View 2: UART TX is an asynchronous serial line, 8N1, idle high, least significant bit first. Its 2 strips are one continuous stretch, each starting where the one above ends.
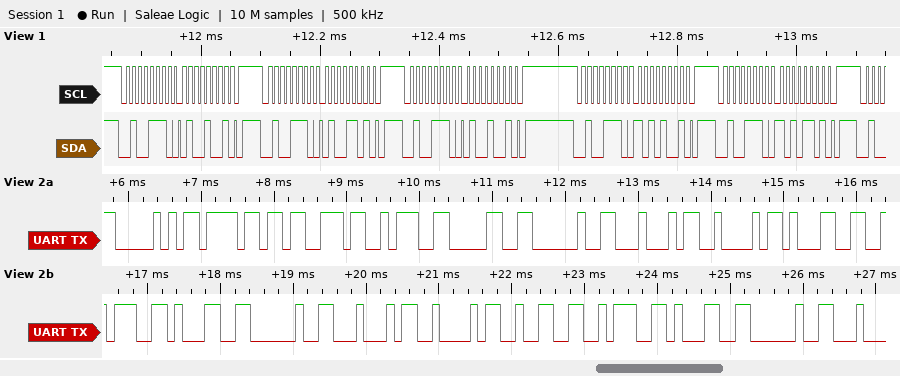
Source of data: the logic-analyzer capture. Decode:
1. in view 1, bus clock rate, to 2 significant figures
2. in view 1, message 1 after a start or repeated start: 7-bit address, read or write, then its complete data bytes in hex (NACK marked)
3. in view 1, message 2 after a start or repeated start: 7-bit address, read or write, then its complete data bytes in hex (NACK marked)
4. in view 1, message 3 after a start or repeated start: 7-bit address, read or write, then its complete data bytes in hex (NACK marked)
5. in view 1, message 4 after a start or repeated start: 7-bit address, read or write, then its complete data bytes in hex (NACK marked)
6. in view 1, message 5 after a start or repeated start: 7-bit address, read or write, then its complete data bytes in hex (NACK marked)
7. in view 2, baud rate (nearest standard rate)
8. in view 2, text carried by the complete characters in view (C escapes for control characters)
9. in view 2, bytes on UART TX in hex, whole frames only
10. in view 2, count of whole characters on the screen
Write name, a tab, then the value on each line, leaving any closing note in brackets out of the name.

in view 1, bus clock rate, to 2 significant figures	100 kHz
in view 1, message 1 after a start or repeated start: 7-bit address, read or write, then its complete data bytes in hex	0x27 write: 49
in view 1, message 2 after a start or repeated start: 7-bit address, read or write, then its complete data bytes in hex	0x27 write: 4D
in view 1, message 3 after a start or repeated start: 7-bit address, read or write, then its complete data bytes in hex	0x27 write: 49
in view 1, message 4 after a start or repeated start: 7-bit address, read or write, then its complete data bytes in hex	0x27 write: A9
in view 1, message 5 after a start or repeated start: 7-bit address, read or write, then its complete data bytes in hex	0x27 write: AD
in view 2, baud rate	9600 baud
in view 2, text carried by the complete characters in view	"Pos:0 DB1:1 DB2:1 "
in view 2, bytes on UART TX in hex, whole frames only	50 6F 73 3A 30 20 44 42 31 3A 31 20 44 42 32 3A 31 20
in view 2, count of whole characters on the screen	18
